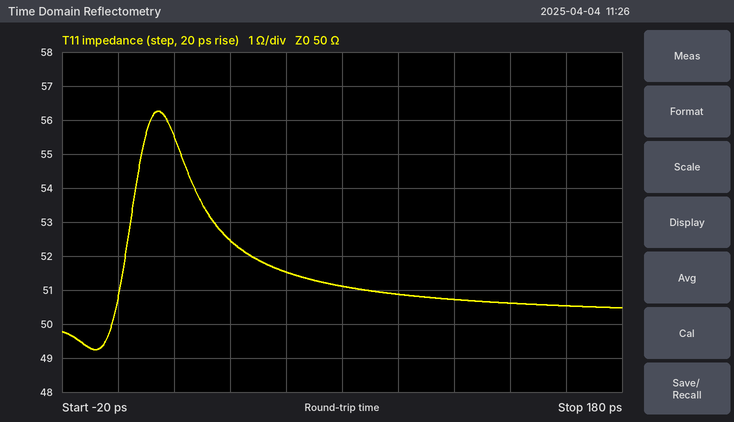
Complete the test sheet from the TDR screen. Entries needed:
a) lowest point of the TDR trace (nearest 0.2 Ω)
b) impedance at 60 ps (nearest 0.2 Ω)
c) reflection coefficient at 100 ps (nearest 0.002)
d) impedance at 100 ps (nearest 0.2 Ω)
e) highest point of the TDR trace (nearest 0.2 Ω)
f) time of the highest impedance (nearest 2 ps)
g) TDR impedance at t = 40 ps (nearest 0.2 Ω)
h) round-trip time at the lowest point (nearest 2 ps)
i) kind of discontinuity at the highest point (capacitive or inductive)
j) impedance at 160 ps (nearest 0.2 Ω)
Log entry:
49.2 Ω
51.6 Ω
+0.008
50.8 Ω
56.2 Ω
14 ps
52.4 Ω
-8 ps
inductive
50.6 Ω
